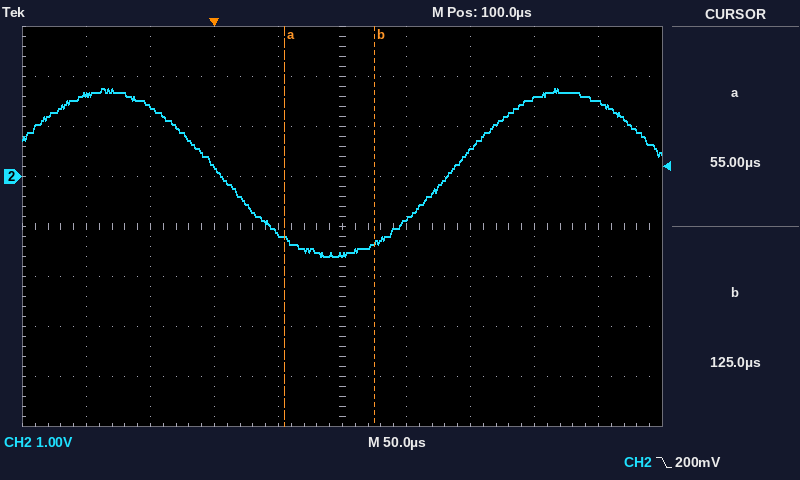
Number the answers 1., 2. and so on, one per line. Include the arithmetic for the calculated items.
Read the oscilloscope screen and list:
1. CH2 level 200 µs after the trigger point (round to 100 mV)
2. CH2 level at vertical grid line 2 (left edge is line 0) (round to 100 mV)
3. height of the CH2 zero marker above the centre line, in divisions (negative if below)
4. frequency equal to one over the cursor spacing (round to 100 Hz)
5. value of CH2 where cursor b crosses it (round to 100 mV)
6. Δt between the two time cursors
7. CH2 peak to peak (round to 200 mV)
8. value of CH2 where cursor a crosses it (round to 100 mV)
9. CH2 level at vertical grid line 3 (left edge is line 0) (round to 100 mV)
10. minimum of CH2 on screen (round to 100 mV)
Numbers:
1. 500 mV
2. 1.4 V
3. +1.0 div
4. 1 / 70 µs ≈ 14.3 kHz
5. -1.3 V
6. 125 µs − (55 µs) = 70 µs
7. 3.4 V
8. -1.2 V
9. 200 mV
10. -1.6 V
